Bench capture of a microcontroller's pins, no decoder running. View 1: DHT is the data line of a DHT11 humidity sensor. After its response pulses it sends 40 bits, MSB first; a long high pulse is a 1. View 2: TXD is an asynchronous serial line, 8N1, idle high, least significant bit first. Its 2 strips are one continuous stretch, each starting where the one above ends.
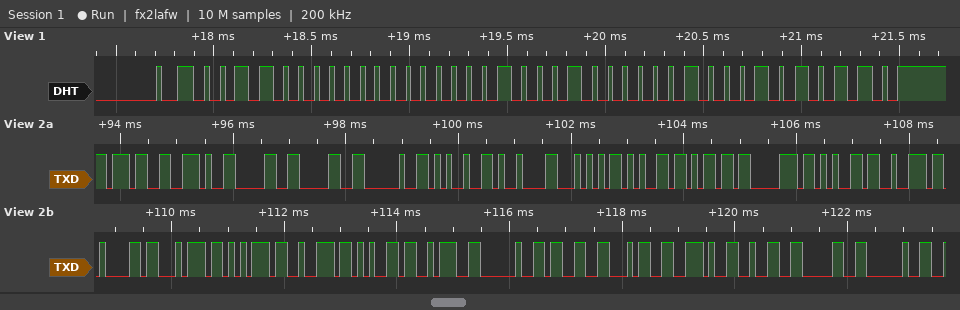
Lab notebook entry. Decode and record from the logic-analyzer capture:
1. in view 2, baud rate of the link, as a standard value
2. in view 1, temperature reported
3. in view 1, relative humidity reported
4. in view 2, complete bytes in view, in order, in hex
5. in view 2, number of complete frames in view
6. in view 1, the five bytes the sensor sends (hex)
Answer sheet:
9600 baud
34.4 °C
48 %
37 2E 30 30 20 25 09 54 65 6D 70 65 72 61 74 75 72 65 3A 20 33 34 2E 32 30 20
26
30 00 22 04 56
